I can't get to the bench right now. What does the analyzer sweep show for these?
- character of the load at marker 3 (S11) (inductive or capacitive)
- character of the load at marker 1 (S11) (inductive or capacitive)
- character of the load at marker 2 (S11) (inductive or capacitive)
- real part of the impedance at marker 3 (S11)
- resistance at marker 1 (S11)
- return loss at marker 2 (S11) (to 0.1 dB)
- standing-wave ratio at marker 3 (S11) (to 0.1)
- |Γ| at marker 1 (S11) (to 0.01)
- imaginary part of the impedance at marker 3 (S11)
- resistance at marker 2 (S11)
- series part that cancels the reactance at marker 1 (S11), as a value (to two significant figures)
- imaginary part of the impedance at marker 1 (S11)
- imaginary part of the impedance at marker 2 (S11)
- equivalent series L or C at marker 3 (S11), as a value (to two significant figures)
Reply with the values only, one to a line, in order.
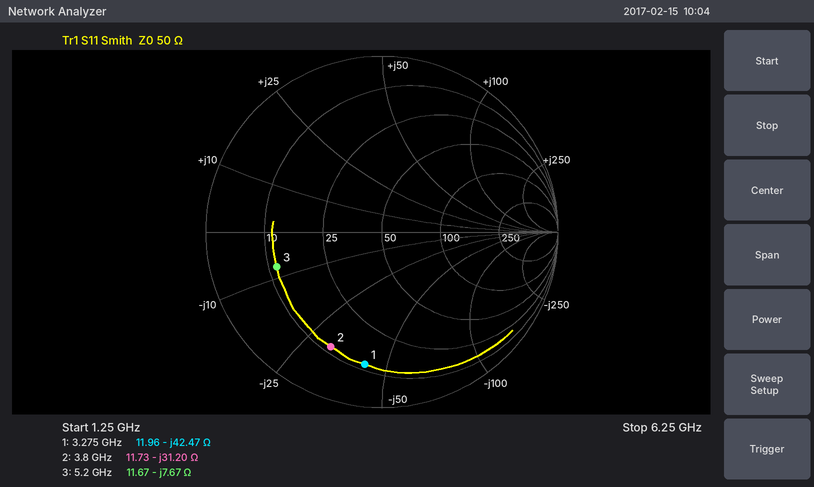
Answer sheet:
capacitive
capacitive
capacitive
11.67 Ω
11.96 Ω
2.9 dB
4.4
0.76
-7.67 Ω
11.73 Ω
2.1 nH
-42.47 Ω
-31.20 Ω
4.0 pF
